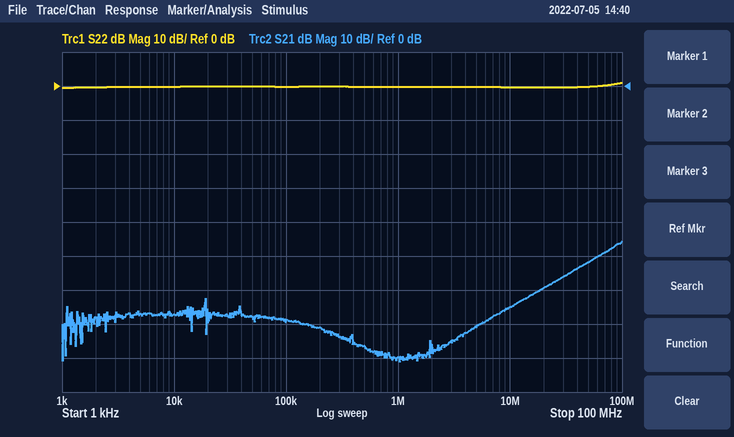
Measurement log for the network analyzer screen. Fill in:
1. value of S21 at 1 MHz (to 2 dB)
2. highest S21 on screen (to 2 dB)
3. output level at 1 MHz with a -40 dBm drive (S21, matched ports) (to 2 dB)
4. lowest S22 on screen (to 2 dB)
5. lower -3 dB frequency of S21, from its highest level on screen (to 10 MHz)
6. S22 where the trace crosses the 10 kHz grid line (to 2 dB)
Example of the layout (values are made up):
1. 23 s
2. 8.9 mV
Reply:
1. -80 dB
2. -46 dB
3. -120 dBm
4. 0 dB
5. 70 MHz
6. 0 dB
